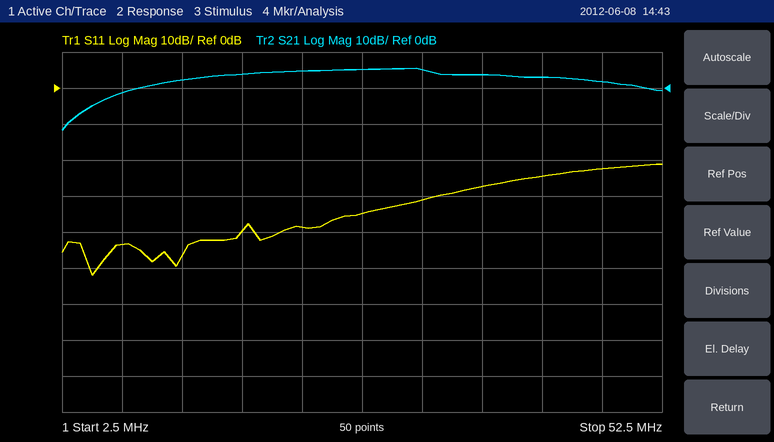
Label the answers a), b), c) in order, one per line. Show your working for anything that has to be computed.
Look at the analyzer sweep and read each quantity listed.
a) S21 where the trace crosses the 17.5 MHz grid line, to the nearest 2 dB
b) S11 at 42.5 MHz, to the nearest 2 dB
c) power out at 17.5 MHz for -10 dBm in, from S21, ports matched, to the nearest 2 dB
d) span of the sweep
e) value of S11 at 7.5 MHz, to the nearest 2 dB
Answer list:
a) 4 dB
b) -24 dB
c) -10 dBm + (4 dB) = -6 dBm
d) 50 MHz
e) -44 dB
